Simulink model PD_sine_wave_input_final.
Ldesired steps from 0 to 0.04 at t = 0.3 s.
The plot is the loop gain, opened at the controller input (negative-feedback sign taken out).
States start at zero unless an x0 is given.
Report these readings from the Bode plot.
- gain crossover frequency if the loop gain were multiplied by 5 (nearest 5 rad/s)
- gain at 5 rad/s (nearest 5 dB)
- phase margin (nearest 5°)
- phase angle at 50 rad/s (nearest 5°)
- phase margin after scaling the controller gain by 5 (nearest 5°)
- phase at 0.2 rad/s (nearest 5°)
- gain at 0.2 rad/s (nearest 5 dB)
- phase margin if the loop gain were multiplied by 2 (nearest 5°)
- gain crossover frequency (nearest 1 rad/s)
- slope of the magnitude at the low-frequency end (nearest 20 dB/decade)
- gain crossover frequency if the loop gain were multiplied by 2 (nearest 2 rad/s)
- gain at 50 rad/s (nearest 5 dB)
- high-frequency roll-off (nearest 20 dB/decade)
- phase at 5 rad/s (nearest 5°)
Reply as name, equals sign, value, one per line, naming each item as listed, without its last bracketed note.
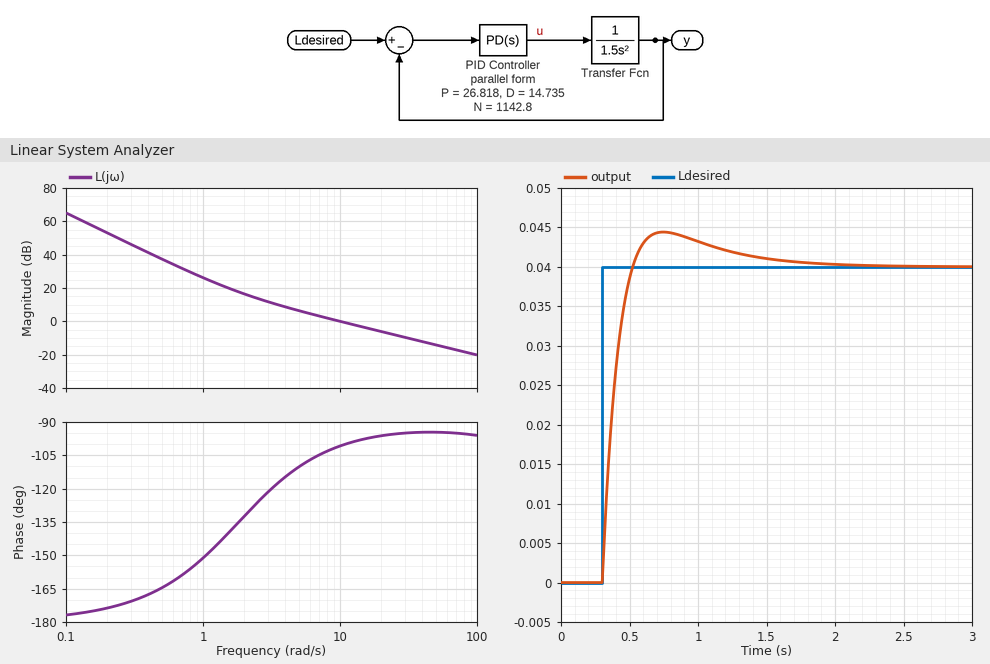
gain crossover frequency if the loop gain were multiplied by 5 = 50 rad/s
gain at 5 rad/s = 5 dB
phase margin = 80°
phase angle at 50 rad/s = -95°
phase margin after scaling the controller gain by 5 = 85°
phase at 0.2 rad/s = -175°
gain at 0.2 rad/s = 55 dB
phase margin if the loop gain were multiplied by 2 = 85°
gain crossover frequency = 10 rad/s
slope of the magnitude at the low-frequency end = -40 dB/decade
gain crossover frequency if the loop gain were multiplied by 2 = 20 rad/s
gain at 50 rad/s = -15 dB
high-frequency roll-off = -20 dB/decade
phase at 5 rad/s = -110°
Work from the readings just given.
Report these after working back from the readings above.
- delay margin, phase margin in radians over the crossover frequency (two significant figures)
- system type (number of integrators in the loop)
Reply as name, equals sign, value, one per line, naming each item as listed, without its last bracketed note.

delay margin, phase margin in radians over the crossover frequency = 0.14 s
system type = 2
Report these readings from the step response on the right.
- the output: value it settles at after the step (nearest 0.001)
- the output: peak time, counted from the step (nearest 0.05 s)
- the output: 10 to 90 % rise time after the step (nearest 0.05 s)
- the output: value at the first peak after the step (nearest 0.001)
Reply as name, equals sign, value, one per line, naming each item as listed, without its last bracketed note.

the output: value it settles at after the step = 0.040
the output: peak time, counted from the step = 0.45 s
the output: 10 to 90 % rise time after the step = 0.15 s
the output: value at the first peak after the step = 0.044
